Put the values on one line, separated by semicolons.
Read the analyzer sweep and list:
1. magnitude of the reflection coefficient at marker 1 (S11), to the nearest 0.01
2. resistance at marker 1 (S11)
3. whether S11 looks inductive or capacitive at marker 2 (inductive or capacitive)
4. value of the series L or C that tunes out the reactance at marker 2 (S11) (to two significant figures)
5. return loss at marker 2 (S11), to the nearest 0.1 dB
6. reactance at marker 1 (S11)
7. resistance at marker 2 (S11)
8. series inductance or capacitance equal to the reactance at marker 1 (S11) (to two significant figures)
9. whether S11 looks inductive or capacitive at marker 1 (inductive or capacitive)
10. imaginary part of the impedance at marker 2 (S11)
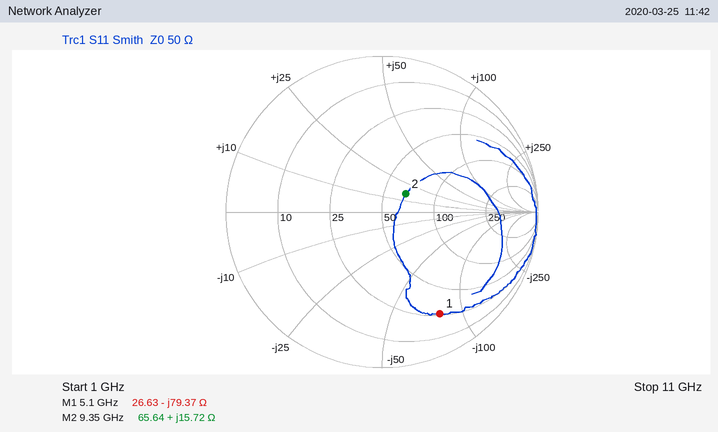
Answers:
0.75; 26.63 Ω; inductive; 1.1 pF; 14.4 dB; -79.37 Ω; 65.64 Ω; 390 fF; capacitive; +15.72 Ω
